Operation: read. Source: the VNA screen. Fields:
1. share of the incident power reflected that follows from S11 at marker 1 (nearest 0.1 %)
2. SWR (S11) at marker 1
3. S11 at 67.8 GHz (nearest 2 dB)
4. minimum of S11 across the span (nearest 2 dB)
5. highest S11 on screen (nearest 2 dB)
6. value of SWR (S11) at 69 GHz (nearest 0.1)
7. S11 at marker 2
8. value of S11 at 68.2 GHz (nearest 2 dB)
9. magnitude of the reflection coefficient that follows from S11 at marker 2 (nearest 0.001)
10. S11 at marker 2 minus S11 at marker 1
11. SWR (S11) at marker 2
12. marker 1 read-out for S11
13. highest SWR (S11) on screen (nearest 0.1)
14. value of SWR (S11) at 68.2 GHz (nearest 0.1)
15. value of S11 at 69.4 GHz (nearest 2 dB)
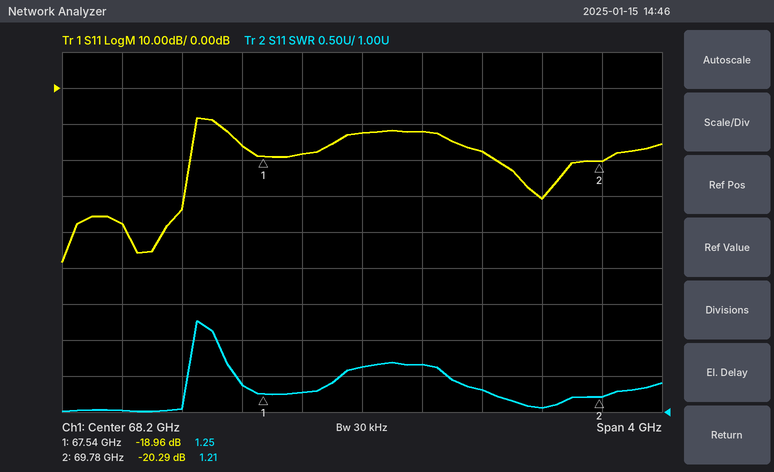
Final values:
1.3 %
1.25
-18 dB
-48 dB
-8 dB
1.3
-20.29 dB
-12 dB
0.097
-1.33 dB
1.21
-18.96 dB
2.3
1.6
-30 dB
